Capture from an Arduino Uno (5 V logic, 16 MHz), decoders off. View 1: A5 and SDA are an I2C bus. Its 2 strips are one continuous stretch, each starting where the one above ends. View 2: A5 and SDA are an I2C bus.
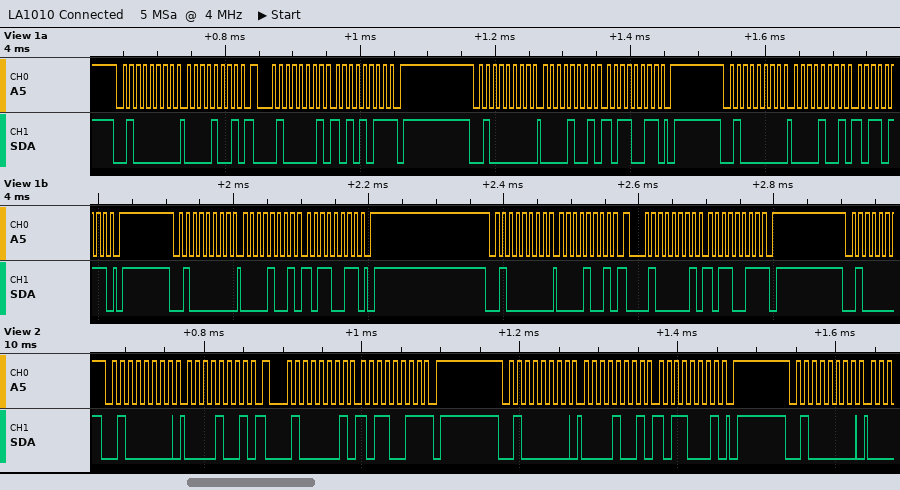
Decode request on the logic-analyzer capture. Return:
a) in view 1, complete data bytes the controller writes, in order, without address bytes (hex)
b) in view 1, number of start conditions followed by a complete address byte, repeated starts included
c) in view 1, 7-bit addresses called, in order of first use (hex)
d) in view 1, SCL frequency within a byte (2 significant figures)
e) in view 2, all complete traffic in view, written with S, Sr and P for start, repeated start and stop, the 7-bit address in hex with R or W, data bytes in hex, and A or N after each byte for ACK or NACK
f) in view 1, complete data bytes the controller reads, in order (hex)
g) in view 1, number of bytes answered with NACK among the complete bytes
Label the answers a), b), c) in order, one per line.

a) 09 09 B3 09 B7 09 B3 09
b) 7
c) 0x20
d) 100 kHz
e) S 20W A 09 A Sr 20R A B3 N P S 20W A 09 A B1 A P S 20W A
f) AB B3
g) 2
